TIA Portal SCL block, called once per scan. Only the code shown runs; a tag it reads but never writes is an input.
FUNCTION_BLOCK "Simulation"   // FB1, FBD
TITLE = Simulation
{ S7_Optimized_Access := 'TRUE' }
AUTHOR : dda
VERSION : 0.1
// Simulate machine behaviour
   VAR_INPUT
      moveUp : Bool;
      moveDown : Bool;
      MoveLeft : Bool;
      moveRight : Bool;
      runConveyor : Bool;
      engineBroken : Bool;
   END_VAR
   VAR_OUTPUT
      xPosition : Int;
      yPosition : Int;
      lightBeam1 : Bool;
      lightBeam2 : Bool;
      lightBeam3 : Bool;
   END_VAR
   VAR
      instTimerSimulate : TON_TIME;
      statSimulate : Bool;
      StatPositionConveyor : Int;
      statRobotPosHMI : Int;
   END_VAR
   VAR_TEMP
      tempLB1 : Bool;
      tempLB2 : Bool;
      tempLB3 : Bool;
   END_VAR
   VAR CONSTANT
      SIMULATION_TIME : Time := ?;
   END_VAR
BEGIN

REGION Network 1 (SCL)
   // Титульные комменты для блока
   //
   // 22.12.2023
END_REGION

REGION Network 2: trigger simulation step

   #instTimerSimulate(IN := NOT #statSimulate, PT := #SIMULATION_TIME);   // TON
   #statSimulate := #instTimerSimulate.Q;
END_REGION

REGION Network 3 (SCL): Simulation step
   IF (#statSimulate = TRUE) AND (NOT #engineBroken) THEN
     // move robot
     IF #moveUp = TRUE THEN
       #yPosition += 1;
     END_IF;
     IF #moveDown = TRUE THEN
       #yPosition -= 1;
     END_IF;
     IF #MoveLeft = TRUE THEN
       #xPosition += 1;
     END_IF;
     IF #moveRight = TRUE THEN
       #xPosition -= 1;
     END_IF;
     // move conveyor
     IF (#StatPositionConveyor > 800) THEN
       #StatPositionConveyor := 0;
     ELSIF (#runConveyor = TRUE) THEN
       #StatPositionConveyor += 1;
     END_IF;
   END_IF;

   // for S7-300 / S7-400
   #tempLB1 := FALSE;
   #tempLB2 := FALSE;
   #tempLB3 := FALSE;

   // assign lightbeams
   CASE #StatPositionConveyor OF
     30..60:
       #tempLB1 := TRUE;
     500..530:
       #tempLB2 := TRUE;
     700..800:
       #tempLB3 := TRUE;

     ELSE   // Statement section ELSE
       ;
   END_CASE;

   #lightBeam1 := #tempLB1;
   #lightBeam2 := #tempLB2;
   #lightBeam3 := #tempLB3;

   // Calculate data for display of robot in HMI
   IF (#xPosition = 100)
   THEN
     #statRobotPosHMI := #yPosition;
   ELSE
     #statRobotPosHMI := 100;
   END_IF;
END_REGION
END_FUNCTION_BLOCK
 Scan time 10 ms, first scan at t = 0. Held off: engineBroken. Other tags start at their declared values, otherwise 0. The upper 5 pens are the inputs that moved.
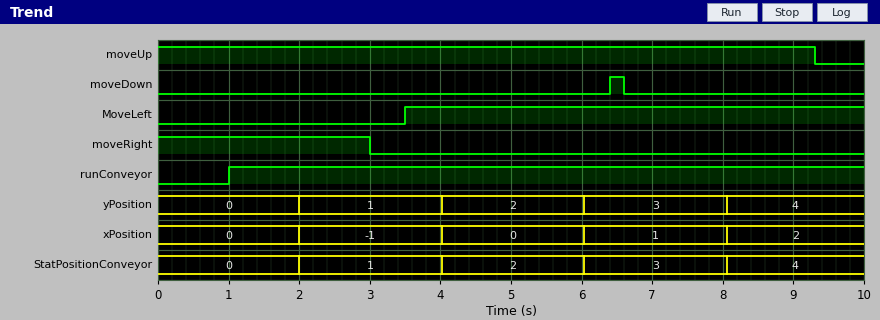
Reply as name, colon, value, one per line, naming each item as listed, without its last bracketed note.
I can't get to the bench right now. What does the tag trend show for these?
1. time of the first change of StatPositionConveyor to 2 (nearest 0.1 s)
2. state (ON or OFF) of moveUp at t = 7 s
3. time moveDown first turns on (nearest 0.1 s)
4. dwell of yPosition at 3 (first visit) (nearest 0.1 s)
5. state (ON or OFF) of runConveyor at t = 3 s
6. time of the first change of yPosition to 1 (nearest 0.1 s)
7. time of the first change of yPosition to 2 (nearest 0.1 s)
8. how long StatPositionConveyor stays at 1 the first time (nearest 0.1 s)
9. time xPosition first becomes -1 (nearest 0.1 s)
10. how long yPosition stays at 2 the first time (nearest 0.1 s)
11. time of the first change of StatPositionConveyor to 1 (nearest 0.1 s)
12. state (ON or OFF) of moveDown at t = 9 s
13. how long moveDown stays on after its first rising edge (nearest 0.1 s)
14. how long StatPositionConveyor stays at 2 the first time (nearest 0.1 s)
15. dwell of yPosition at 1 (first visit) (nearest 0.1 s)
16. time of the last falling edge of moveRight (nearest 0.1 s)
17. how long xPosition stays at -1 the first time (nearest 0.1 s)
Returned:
time of the first change of StatPositionConveyor to 2: 4.0 s
state (ON or OFF) of moveUp at t = 7 s: ON
time moveDown first turns on: 6.4 s
dwell of yPosition at 3 (first visit): 2.0 s
state (ON or OFF) of runConveyor at t = 3 s: ON
time of the first change of yPosition to 1: 2.0 s
time of the first change of yPosition to 2: 4.0 s
how long StatPositionConveyor stays at 1 the first time: 2.0 s
time xPosition first becomes -1: 2.0 s
how long yPosition stays at 2 the first time: 2.0 s
time of the first change of StatPositionConveyor to 1: 2.0 s
state (ON or OFF) of moveDown at t = 9 s: OFF
how long moveDown stays on after its first rising edge: 0.2 s
how long StatPositionConveyor stays at 2 the first time: 2.0 s
dwell of yPosition at 1 (first visit): 2.0 s
time of the last falling edge of moveRight: 3.0 s
how long xPosition stays at -1 the first time: 2.0 s
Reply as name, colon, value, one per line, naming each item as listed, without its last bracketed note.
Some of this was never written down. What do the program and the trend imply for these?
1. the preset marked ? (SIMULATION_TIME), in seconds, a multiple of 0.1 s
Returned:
the preset marked ? (SIMULATION_TIME), in seconds, a multiple of 0.1 s: 2.0 s
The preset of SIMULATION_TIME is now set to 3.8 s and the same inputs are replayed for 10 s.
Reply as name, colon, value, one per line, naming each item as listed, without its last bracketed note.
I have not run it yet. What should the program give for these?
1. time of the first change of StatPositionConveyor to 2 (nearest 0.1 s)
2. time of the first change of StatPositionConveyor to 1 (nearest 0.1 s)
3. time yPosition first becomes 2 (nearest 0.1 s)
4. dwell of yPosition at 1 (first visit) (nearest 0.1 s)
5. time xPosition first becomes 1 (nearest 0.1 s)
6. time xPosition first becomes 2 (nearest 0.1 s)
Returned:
time of the first change of StatPositionConveyor to 2: 7.6 s
time of the first change of StatPositionConveyor to 1: 3.8 s
time yPosition first becomes 2: 7.6 s
dwell of yPosition at 1 (first visit): 3.8 s
time xPosition first becomes 1: 3.8 s
time xPosition first becomes 2: 7.6 s
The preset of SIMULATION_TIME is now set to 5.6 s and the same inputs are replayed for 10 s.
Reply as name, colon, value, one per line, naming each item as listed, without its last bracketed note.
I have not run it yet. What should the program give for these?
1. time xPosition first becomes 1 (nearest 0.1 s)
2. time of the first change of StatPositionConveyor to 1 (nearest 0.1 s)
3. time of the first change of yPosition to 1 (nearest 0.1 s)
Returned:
time xPosition first becomes 1: 5.6 s
time of the first change of StatPositionConveyor to 1: 5.6 s
time of the first change of yPosition to 1: 5.6 s
